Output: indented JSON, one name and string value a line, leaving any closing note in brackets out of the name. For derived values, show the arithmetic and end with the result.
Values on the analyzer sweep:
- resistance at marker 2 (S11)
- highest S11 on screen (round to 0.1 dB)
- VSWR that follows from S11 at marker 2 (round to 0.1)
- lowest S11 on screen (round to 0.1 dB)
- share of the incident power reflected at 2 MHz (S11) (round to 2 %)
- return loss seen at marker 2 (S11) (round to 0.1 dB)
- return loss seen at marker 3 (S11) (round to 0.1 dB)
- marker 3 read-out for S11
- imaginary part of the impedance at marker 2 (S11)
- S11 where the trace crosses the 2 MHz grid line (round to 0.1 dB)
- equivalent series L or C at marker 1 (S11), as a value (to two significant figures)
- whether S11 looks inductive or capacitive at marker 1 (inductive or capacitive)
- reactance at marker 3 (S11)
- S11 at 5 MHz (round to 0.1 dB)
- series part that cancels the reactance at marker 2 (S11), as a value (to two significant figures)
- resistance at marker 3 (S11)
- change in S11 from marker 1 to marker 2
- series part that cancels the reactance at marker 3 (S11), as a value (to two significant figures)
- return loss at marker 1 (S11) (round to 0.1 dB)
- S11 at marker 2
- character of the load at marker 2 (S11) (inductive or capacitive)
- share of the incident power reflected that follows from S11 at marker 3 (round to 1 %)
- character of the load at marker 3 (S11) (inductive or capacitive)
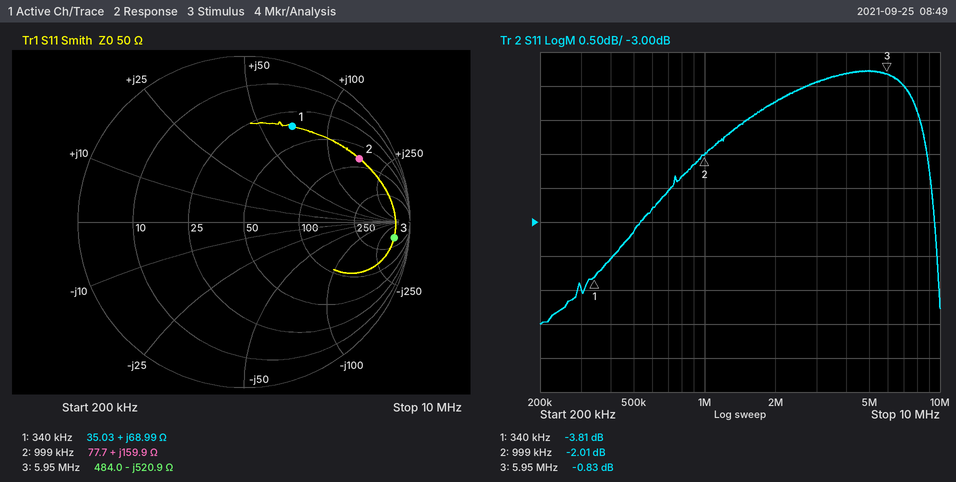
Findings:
{
  "resistance at marker 2": "77.7 Ω",
  "highest S11 on screen": "-0.8 dB",
  "VSWR that follows from S11 at marker 2": "(1 + 0.7934)/(1 − 0.7934) ≈ 8.7",
  "lowest S11 on screen": "-4.5 dB",
  "share of the incident power reflected at 2 MHz (S11)": "10^(-1.2/10) ≈ 76 %",
  "return loss seen at marker 2 (S11)": "2.0 dB",
  "return loss seen at marker 3 (S11)": "0.8 dB",
  "marker 3 read-out for S11": "-0.83 dB",
  "imaginary part of the impedance at marker 2": "+159.9 Ω",
  "S11 where the trace crosses the 2 MHz grid line": "-1.2 dB",
  "equivalent series L or C at marker 1 (S11), as a value": "L = 68.99 Ω/(2π × 340 kHz) ≈ 32 µH",
  "whether S11 looks inductive or capacitive at marker 1": "inductive",
  "reactance at marker 3": "-520.9 Ω",
  "S11 at 5 MHz": "-0.8 dB",
  "series part that cancels the reactance at marker 2 (S11), as a value": "C = 1/(2π × 999 kHz × 159.9 Ω) ≈ 1.00 nF",
  "resistance at marker 3": "484.0 Ω",
  "change in S11 from marker 1 to marker 2": "-2.01 − (-3.81) = 1.80 dB",
  "series part that cancels the reactance at marker 3 (S11), as a value": "L = 520.9 Ω/(2π × 5.95 MHz) ≈ 14 µH",
  "return loss at marker 1 (S11)": "3.8 dB",
  "S11 at marker 2": "-2.01 dB",
  "character of the load at marker 2 (S11)": "inductive",
  "share of the incident power reflected that follows from S11 at marker 3": "10^(-0.83/10) ≈ 83 %",
  "character of the load at marker 3 (S11)": "capacitive"
}
